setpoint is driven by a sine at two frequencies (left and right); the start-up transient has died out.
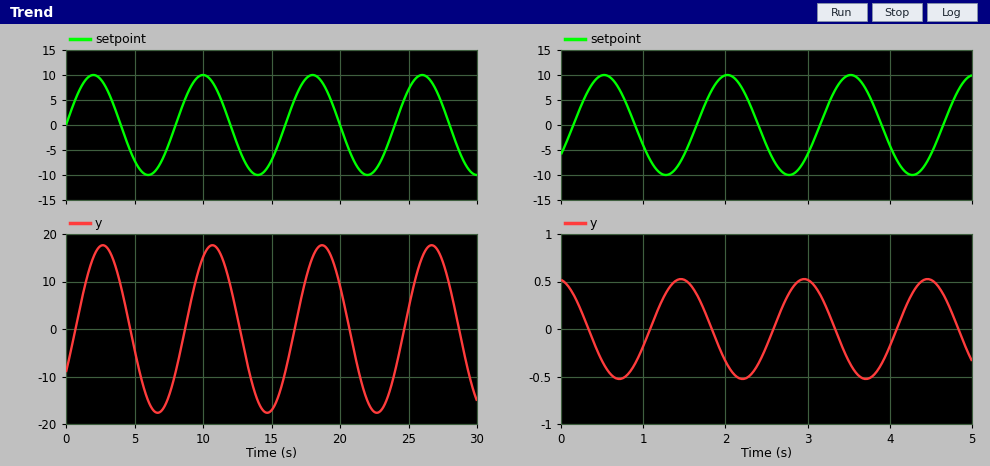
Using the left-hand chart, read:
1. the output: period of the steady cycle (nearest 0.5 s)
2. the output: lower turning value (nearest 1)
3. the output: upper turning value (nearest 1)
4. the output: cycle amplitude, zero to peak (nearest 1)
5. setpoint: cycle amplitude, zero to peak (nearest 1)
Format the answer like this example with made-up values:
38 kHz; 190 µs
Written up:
8.0 s; -18; 18; 18; 10
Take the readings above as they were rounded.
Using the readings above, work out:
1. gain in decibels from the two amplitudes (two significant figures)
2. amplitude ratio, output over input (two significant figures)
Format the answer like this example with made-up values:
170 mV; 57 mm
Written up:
5.1 dB; 1.8
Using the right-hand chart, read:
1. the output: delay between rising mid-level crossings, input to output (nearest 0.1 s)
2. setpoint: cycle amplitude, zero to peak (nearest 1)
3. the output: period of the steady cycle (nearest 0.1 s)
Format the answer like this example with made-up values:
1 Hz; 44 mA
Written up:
0.9 s; 10; 1.5 s
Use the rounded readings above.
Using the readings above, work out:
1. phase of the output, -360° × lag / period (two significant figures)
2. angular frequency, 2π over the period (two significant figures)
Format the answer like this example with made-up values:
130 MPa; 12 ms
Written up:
-220°; 4.2 rad/s
